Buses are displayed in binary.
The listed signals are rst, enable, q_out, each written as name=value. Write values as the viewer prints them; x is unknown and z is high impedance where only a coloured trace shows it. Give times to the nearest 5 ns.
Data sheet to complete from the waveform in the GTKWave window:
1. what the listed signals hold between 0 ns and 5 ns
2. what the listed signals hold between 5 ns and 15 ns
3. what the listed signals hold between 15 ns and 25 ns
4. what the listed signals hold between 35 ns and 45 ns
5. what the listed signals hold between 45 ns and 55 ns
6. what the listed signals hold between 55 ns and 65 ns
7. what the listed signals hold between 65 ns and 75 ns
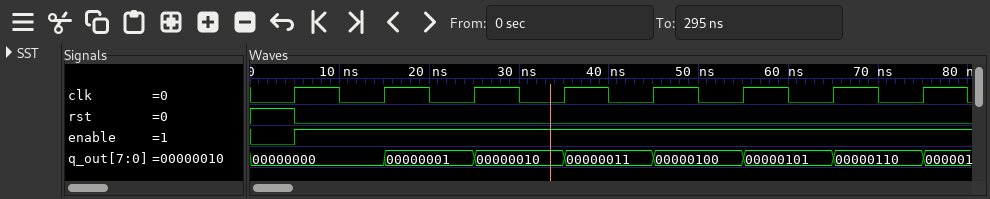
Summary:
rst=1, enable=0, q_out=00000000
rst=0, enable=1, q_out=00000000
rst=0, enable=1, q_out=00000001
rst=0, enable=1, q_out=00000011
rst=0, enable=1, q_out=00000100
rst=0, enable=1, q_out=00000101
rst=0, enable=1, q_out=00000110
